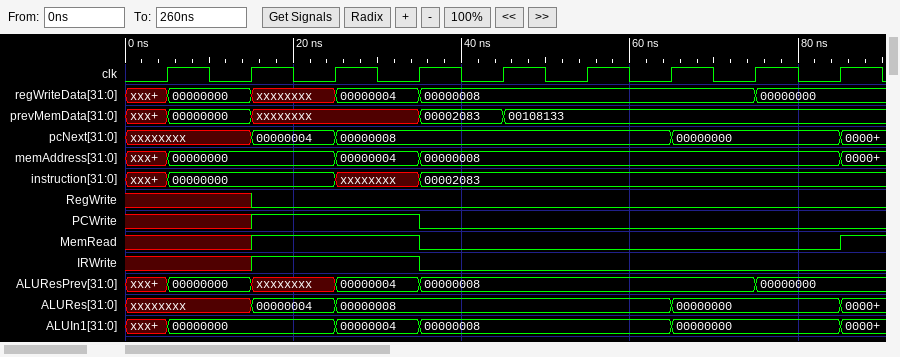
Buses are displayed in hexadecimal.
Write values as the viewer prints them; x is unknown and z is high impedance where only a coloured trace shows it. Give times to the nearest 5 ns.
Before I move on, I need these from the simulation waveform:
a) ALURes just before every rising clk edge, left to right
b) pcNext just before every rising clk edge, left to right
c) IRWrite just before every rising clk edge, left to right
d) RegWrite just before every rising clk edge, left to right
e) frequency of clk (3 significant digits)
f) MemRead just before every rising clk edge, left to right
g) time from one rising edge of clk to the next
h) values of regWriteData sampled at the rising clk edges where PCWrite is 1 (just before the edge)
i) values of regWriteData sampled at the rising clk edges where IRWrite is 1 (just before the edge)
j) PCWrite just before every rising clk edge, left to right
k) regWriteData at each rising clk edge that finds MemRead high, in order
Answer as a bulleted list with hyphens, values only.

- xxxxxxxx, xxxxxxxx, 00000004, 00000008, 00000008, 00000008, 00000008, 00000000, 00000000
- xxxxxxxx, xxxxxxxx, 00000004, 00000008, 00000008, 00000008, 00000008, 00000000, 00000000
- x x 1 1 0 0 0 0 0
- x x 0 0 0 0 0 0 0
- 100 MHz
- x x 1 1 0 0 0 0 0
- 10 ns
- xxxxxxxx, 00000004
- xxxxxxxx, 00000004
- x x 1 1 0 0 0 0 0
- xxxxxxxx, 00000004
